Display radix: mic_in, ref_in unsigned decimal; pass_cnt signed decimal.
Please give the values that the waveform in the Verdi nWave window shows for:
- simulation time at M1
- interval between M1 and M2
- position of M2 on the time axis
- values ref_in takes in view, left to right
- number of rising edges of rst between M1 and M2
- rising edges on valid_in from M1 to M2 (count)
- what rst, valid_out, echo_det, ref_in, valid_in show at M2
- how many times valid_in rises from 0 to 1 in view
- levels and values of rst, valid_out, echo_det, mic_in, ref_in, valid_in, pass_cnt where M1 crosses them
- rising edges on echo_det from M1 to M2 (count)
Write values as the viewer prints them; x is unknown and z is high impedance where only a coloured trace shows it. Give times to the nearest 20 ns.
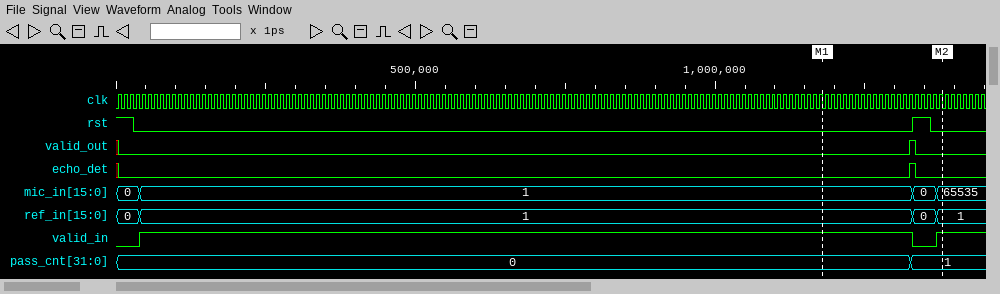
1180 ns
200 ns
1380 ns
0, 1, 0, 1
1
1
rst=0, valid_out=0, echo_det=0, ref_in=1, valid_in=1
2
rst=0, valid_out=0, echo_det=0, mic_in=1, ref_in=1, valid_in=1, pass_cnt=0
1
